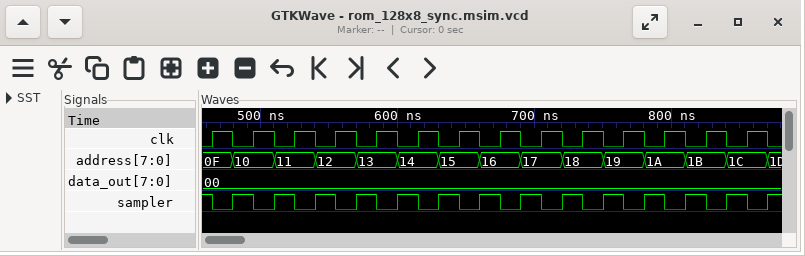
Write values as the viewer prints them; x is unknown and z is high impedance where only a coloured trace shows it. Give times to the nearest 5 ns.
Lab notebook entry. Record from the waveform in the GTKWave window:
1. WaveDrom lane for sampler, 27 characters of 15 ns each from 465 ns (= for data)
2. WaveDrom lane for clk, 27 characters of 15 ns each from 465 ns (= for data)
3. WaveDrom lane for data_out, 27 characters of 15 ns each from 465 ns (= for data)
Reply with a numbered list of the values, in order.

1. {name: 'sampler', wave: '010101010101010101010101010'}
2. {name: 'clk', wave: '101010101010101010101010101'}
3. {name: 'data_out', wave: '=..........................', data: '00'}
